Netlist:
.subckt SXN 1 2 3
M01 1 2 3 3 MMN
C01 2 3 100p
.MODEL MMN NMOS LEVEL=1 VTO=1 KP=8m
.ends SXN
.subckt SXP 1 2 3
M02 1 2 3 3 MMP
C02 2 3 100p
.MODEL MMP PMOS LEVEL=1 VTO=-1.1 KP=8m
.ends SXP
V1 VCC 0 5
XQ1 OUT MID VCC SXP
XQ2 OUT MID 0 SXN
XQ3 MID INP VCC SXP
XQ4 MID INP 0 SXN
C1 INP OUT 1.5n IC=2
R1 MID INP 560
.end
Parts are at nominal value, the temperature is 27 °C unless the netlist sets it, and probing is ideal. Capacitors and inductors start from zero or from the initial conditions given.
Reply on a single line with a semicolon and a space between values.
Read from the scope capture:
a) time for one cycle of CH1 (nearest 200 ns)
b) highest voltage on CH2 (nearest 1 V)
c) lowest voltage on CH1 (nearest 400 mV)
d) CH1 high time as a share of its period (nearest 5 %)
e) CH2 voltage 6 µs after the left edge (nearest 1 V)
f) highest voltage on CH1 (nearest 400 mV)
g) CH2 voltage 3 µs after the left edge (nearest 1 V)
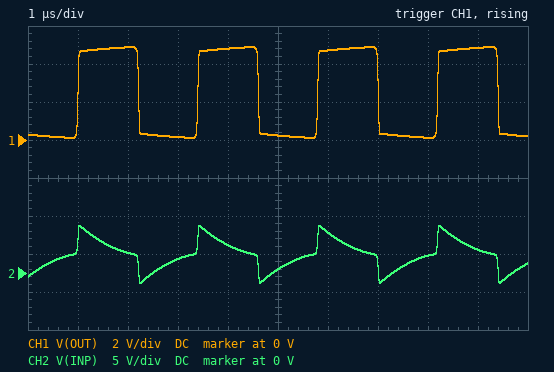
2.4 µs; 6 V; 0 V; 50 %; 5 V; 4.8 V; 2 V
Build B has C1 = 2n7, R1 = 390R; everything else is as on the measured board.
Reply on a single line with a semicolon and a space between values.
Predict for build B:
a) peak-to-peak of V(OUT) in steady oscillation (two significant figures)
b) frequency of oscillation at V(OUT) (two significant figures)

4.7 V; 340 kHz
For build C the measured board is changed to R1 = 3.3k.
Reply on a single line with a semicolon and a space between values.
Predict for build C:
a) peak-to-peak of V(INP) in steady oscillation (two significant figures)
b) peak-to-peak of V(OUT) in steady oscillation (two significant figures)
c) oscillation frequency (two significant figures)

8.6 V; 5.0 V; 80 kHz
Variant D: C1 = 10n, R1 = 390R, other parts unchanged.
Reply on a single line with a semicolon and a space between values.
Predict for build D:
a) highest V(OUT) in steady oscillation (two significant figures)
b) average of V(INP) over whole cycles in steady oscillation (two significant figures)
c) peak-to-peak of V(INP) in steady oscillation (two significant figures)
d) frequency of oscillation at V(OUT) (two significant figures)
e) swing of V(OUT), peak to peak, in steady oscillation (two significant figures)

4.8 V; 2.5 V; 8.0 V; 100 kHz; 4.6 V
